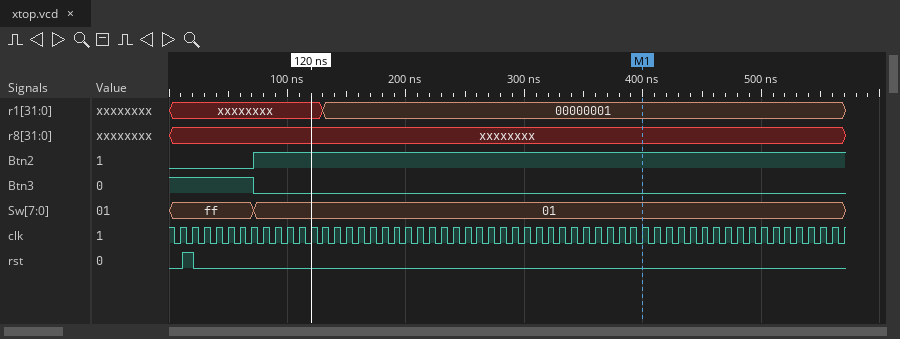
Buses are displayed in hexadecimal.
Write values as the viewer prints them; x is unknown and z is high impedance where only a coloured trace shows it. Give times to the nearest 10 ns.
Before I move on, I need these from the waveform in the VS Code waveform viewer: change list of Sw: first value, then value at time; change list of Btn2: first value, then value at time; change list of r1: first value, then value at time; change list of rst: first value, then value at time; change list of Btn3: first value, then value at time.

ff, 01 at 70 ns
0, 1 at 70 ns
xxxxxxxx, 00000001 at 130 ns
0, 1 at 10 ns, 0 at 20 ns
1, 0 at 70 ns
